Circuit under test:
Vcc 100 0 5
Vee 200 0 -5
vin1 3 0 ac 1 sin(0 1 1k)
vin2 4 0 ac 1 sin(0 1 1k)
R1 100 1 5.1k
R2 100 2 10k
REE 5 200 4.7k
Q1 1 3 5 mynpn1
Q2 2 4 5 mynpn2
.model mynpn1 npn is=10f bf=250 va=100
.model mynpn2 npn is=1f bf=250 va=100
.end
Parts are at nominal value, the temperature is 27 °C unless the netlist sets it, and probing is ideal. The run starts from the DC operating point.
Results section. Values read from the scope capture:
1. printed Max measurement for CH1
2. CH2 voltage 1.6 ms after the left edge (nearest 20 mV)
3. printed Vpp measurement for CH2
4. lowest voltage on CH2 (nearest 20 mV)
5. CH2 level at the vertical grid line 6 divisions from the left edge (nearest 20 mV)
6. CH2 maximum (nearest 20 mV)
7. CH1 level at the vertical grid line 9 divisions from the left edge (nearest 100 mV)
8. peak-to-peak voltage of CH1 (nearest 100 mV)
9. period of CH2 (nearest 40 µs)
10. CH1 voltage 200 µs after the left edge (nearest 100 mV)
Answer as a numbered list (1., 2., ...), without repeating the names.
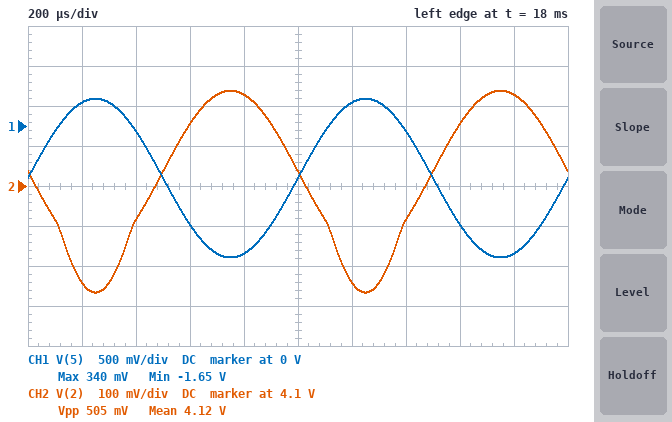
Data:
1. 340 mV
2. 4.26 V
3. 505 mV
4. 3.84 V
5. 3.86 V
6. 4.34 V
7. -1.6 V
8. 2.0 V
9. 1.00 ms
10. 300 mV
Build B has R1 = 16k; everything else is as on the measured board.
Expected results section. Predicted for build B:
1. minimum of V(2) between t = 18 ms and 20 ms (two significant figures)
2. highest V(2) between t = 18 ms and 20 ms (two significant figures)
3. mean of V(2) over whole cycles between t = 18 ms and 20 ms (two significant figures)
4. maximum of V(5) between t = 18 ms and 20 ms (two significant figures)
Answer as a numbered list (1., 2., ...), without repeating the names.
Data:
1. 3.3 V
2. 4.1 V
3. 3.7 V
4. 330 mV
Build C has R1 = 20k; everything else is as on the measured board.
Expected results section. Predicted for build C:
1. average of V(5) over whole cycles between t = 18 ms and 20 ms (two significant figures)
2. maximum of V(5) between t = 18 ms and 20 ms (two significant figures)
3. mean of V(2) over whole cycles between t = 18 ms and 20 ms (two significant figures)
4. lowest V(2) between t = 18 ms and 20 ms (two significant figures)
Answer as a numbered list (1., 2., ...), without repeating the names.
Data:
1. -660 mV
2. 330 mV
3. 3.7 V
4. 3.3 V
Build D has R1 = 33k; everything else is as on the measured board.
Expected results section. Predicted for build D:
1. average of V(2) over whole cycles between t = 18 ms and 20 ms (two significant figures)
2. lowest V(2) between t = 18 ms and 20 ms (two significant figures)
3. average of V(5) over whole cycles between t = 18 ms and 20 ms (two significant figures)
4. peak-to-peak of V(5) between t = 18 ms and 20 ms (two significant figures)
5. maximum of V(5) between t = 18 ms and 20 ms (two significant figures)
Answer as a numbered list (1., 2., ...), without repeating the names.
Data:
1. 3.6 V
2. 3.2 V
3. -660 mV
4. 2.0 V
5. 330 mV
